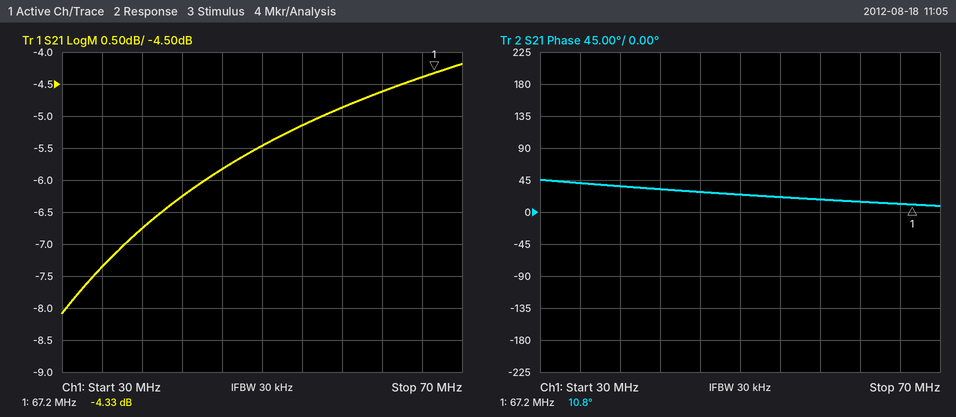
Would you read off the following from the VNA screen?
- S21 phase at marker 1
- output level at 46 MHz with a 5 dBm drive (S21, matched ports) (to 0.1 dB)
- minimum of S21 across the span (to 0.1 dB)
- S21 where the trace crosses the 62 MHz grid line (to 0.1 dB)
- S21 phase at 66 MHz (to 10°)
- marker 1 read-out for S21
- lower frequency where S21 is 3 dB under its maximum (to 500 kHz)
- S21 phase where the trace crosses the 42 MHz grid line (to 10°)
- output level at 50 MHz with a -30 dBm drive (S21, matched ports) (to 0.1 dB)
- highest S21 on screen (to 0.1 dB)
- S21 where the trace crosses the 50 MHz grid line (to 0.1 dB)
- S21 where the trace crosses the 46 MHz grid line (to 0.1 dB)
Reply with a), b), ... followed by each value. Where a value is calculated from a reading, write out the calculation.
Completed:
a) 10.8°
b) 5 dBm + (-5.8 dB) = -0.8 dBm
c) -8.1 dB
d) -4.6 dB
e) 10°
f) -4.33 dB
g) 35.0 MHz
h) 30°
i) -30 dBm + (-5.5 dB) = -35.5 dBm
j) -4.2 dB
k) -5.5 dB
l) -5.8 dB
